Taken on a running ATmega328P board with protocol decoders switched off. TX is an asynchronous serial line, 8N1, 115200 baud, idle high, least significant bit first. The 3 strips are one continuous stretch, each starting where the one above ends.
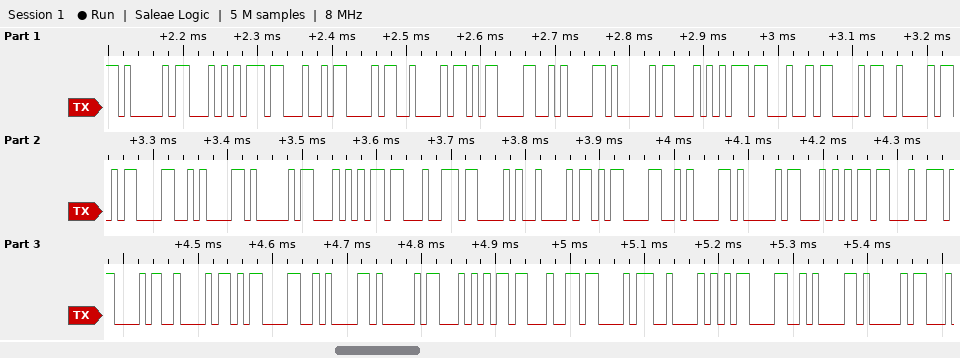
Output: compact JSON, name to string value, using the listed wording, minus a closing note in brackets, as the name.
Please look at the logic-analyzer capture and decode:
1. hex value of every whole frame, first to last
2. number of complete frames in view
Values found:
{"hex value of every whole frame, first to last": "41 54 23 43 42 0D 0A 41 54 23 43 42 0D 0A 41 54 23 43 42 0D 0A 41 54 23 43 42 0D 0A 41 54 23 43 42 0D 0A 41", "number of complete frames in view": "36"}
